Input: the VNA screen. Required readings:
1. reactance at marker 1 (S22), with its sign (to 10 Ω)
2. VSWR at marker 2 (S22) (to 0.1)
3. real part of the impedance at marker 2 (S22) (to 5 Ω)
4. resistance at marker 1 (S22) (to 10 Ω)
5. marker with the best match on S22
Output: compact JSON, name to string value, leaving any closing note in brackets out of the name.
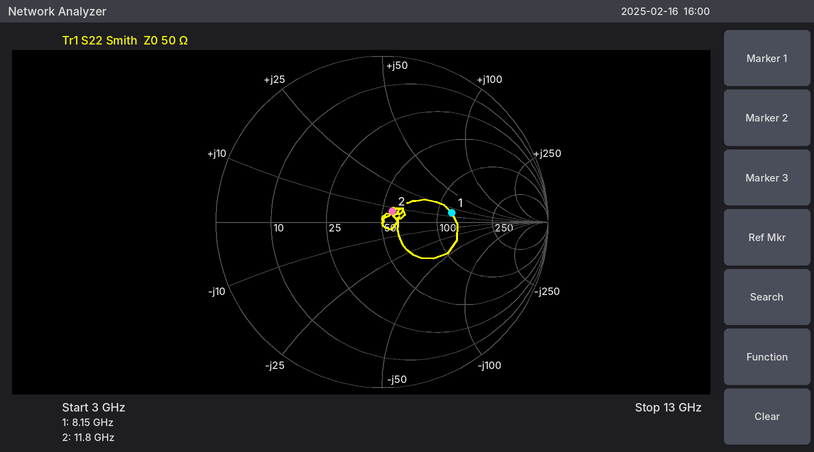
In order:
{"reactance at marker 1 (S22), with its sign": "+20 Ω", "VSWR at marker 2 (S22)": "1.2", "real part of the impedance at marker 2 (S22)": "55 Ω", "resistance at marker 1 (S22)": "120 Ω", "marker with the best match on S22": "marker 2"}
